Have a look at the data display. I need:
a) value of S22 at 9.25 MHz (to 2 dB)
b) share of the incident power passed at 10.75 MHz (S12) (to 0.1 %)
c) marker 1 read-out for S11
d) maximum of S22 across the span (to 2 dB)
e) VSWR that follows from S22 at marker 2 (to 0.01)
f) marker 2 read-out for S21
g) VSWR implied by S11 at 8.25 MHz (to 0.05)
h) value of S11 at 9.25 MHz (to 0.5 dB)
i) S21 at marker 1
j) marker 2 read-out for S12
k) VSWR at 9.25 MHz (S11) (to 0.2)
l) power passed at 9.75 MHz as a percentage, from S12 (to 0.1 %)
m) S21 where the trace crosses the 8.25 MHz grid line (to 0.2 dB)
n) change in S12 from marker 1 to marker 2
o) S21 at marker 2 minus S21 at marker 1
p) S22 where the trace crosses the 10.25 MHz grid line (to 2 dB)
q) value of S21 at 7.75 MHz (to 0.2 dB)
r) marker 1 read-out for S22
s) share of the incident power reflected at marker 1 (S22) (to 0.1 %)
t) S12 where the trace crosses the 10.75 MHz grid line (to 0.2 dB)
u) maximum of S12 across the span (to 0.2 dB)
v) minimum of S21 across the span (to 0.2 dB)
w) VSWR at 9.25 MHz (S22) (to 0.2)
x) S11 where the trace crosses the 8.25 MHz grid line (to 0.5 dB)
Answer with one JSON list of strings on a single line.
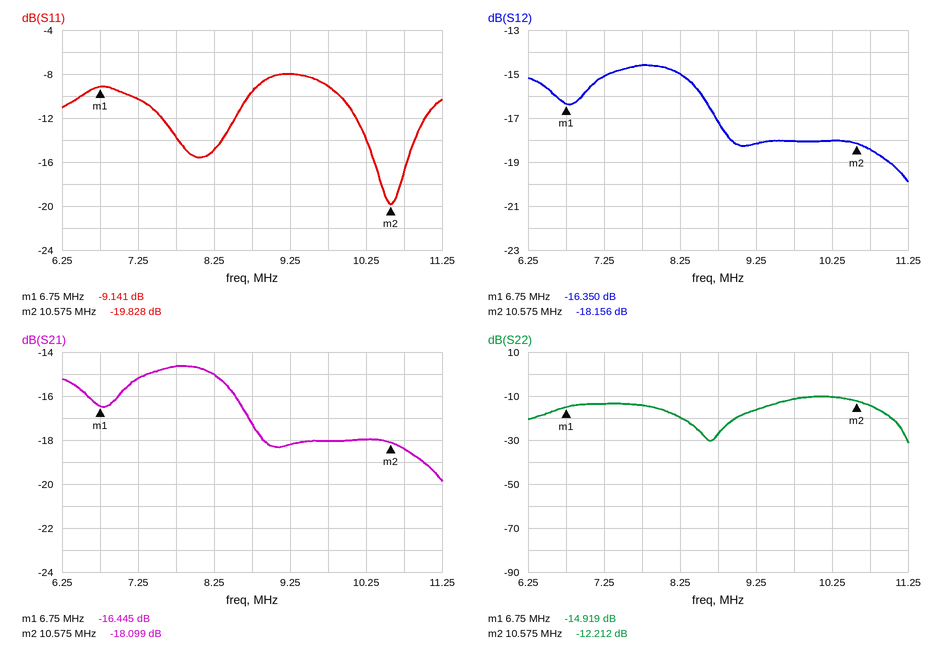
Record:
["-16 dB", "1.4 %", "-9.141 dB", "-10 dB", "1.65", "-18.099 dB", "1.45", "-8.0 dB", "-16.445 dB", "-18.156 dB", "2.4", "1.6 %", "-15.0 dB", "-1.806 dB", "-1.654 dB", "-10 dB", "-14.6 dB", "-14.919 dB", "3.2 %", "-18.4 dB", "-14.6 dB", "-19.8 dB", "1.4", "-15.0 dB"]
